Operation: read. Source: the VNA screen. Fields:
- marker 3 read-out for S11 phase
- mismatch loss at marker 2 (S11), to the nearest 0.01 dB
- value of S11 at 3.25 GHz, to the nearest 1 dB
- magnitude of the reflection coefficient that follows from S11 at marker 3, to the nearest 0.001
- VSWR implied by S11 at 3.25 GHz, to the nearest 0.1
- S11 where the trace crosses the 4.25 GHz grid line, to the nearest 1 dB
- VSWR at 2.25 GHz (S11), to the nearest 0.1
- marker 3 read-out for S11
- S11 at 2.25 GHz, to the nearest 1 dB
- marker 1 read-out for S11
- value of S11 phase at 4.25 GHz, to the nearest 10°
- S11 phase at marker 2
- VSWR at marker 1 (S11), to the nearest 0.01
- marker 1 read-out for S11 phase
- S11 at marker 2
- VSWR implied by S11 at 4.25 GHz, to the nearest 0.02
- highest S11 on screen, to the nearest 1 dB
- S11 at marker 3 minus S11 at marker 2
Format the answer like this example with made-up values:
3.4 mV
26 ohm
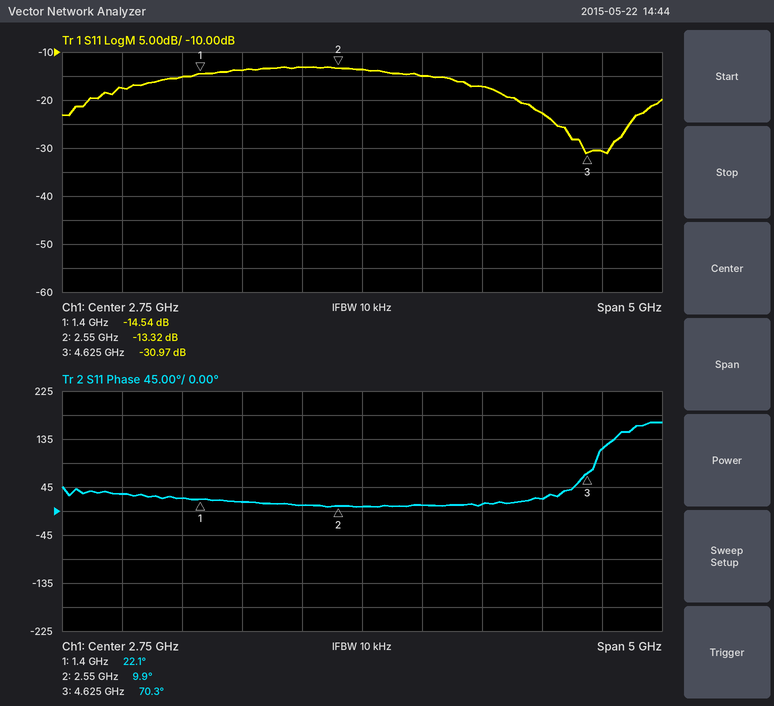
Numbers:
70.3°
0.21 dB
-15 dB
0.028
1.4
-23 dB
1.6
-30.97 dB
-13 dB
-14.54 dB
20°
9.9°
1.46
22.1°
-13.32 dB
1.16
-13 dB
-17.65 dB
